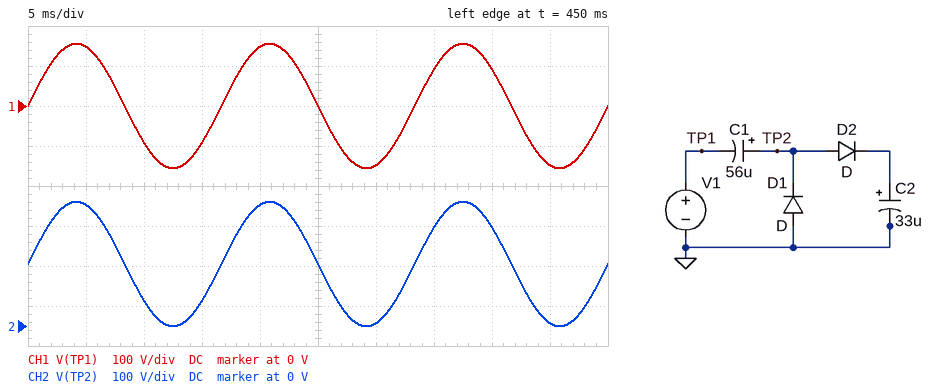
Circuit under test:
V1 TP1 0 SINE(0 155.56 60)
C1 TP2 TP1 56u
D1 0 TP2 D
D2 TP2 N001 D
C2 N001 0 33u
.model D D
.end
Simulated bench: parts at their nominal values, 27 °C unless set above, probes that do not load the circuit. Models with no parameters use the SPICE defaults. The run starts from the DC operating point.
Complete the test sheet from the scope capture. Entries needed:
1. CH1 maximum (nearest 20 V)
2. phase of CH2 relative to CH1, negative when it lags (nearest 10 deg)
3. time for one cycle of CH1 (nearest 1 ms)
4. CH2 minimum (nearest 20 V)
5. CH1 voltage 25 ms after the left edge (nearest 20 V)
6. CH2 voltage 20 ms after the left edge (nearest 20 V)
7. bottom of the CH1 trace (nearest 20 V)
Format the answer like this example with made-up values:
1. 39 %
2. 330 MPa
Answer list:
1. 160 V
2. 0 deg
3. 17 ms
4. 0 V
5. 0 V
6. 300 V
7. -160 V
